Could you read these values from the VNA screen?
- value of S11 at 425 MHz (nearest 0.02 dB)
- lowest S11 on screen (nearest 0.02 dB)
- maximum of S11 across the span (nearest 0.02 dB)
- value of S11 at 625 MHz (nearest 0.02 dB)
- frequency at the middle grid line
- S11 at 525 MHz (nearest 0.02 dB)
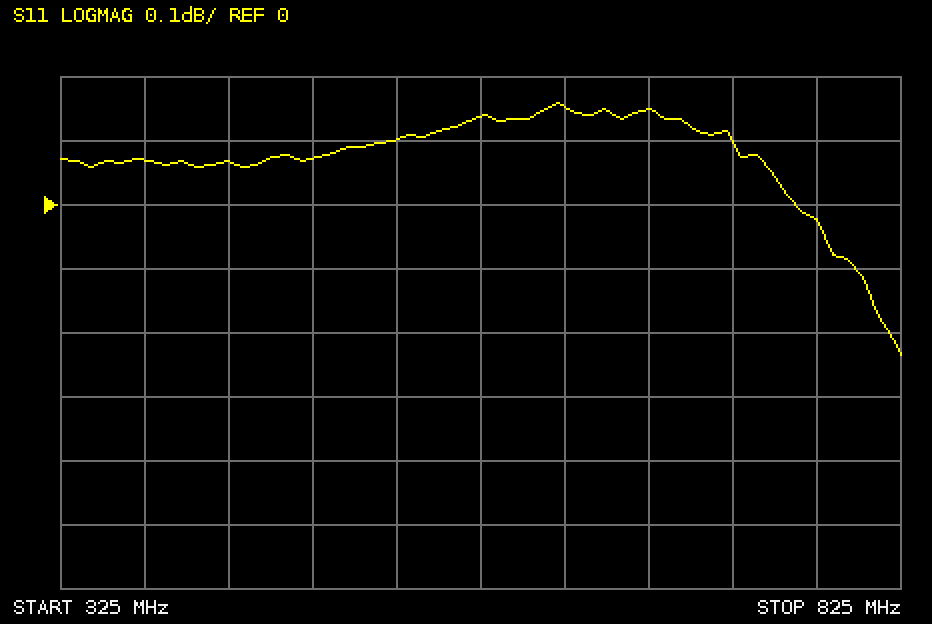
0.06 dB
-0.24 dB
0.16 dB
0.16 dB
575 MHz
0.10 dB
